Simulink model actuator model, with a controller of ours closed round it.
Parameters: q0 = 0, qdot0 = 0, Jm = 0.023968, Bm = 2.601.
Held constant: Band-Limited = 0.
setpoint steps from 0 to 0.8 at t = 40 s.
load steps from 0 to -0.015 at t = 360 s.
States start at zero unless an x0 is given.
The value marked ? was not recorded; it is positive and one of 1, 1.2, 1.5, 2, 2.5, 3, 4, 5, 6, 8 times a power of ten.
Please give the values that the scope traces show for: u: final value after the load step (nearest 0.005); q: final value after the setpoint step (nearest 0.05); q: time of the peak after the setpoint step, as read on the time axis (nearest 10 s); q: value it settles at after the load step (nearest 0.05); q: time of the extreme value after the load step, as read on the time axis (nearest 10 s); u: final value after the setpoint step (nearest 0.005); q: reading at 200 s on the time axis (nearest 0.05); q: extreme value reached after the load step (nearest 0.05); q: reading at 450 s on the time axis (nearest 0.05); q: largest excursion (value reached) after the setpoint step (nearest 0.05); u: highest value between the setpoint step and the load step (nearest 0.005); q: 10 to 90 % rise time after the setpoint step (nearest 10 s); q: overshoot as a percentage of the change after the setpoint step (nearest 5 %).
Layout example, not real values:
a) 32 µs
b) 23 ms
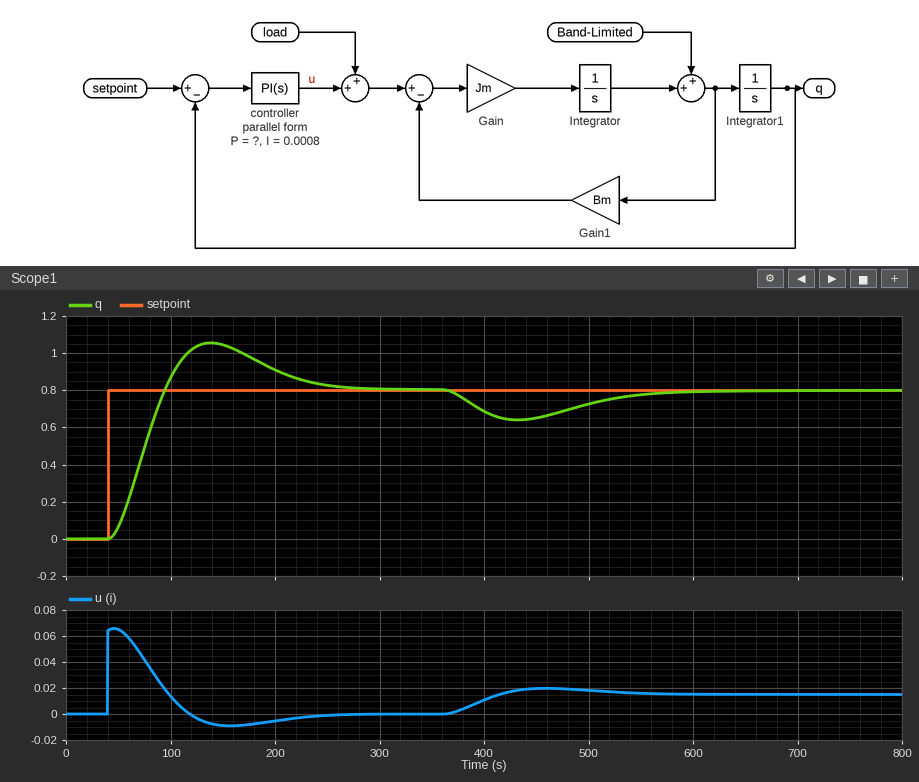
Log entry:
a) 0.015
b) 0.80
c) 140 s
d) 0.80
e) 430 s
f) 0.000
g) 0.90
h) 0.65
i) 0.65
j) 1.05
k) 0.065
l) 40 s
m) 30 %
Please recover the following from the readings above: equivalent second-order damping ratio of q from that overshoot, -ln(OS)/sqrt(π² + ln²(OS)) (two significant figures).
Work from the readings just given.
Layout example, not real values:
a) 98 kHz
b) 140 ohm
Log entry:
a) 0.36
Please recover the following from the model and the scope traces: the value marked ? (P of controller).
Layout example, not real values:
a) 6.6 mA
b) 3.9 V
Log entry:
a) 0.08
